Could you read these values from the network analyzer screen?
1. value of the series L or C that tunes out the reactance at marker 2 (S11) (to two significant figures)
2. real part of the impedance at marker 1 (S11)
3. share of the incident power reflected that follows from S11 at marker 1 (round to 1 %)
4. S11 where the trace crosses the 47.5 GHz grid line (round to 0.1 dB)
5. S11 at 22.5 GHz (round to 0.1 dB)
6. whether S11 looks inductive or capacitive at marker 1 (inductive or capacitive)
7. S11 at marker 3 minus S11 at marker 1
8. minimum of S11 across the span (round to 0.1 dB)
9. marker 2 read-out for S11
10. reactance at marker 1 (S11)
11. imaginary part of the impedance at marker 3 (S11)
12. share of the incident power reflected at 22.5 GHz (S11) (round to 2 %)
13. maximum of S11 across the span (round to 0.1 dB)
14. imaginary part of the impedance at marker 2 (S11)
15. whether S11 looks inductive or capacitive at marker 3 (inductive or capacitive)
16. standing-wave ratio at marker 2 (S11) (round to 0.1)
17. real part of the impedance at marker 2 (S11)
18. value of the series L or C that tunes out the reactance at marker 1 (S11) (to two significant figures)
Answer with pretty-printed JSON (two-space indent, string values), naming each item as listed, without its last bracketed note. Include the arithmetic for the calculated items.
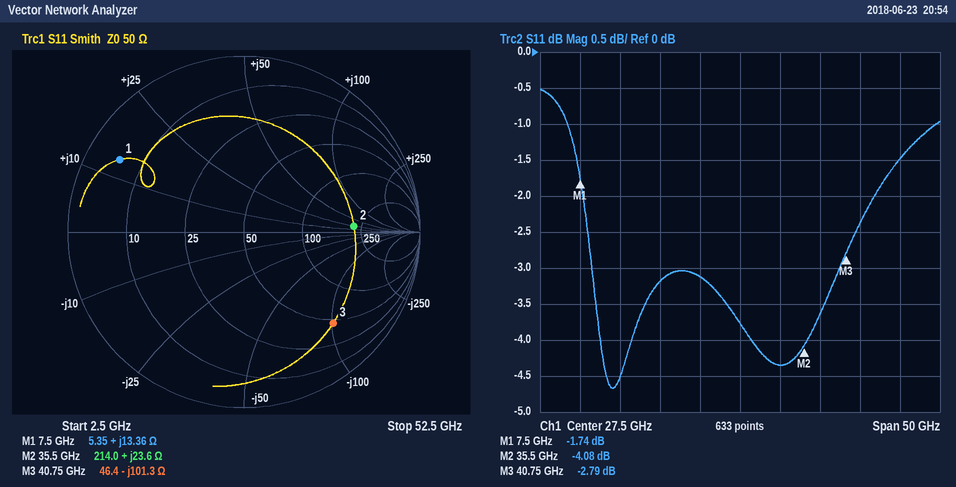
{
  "value of the series L or C that tunes out the reactance at marker 2 (S11)": "C = 1/(2π × 35.5 GHz × 23.6 Ω) ≈ 190 fF",
  "real part of the impedance at marker 1": "5.35 Ω",
  "share of the incident power reflected that follows from S11 at marker 1": "10^(-1.74/10) ≈ 67 %",
  "S11 where the trace crosses the 47.5 GHz grid line": "-1.5 dB",
  "S11 at 22.5 GHz": "-3.1 dB",
  "whether S11 looks inductive or capacitive at marker 1": "inductive",
  "S11 at marker 3 minus S11 at marker 1": "-2.79 − (-1.74) = -1.05 dB",
  "minimum of S11 across the span": "-4.7 dB",
  "marker 2 read-out for S11": "-4.08 dB",
  "reactance at marker 1": "+13.36 Ω",
  "imaginary part of the impedance at marker 3": "-101.3 Ω",
  "share of the incident power reflected at 22.5 GHz (S11)": "10^(-3.1/10) ≈ 49.0 %, so 48 % to the nearest 2 %",
  "maximum of S11 across the span": "-0.5 dB",
  "imaginary part of the impedance at marker 2": "+23.6 Ω",
  "whether S11 looks inductive or capacitive at marker 3": "capacitive",
  "standing-wave ratio at marker 2 (S11)": "4.3",
  "real part of the impedance at marker 2": "214.0 Ω",
  "value of the series L or C that tunes out the reactance at marker 1 (S11)": "C = 1/(2π × 7.5 GHz × 13.36 Ω) ≈ 1.6 pF"
}
